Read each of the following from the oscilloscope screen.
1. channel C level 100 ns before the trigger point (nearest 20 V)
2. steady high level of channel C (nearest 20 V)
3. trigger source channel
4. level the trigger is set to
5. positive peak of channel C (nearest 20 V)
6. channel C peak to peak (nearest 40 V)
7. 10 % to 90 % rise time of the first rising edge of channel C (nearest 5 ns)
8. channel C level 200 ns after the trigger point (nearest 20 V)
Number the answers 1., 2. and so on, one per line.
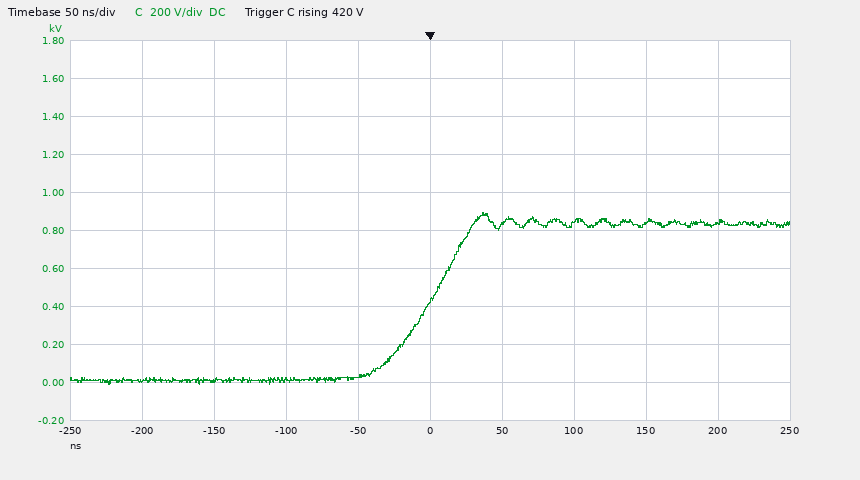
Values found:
1. 20 V
2. 840 V
3. channel C
4. 420 V
5. 900 V
6. 920 V
7. 55 ns
8. 840 V
